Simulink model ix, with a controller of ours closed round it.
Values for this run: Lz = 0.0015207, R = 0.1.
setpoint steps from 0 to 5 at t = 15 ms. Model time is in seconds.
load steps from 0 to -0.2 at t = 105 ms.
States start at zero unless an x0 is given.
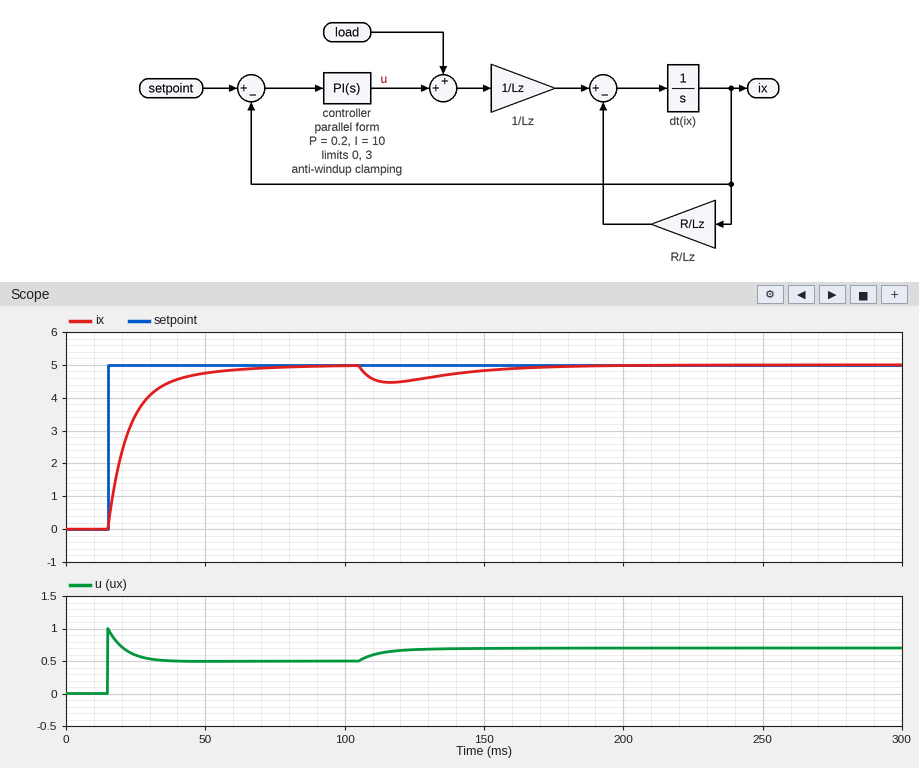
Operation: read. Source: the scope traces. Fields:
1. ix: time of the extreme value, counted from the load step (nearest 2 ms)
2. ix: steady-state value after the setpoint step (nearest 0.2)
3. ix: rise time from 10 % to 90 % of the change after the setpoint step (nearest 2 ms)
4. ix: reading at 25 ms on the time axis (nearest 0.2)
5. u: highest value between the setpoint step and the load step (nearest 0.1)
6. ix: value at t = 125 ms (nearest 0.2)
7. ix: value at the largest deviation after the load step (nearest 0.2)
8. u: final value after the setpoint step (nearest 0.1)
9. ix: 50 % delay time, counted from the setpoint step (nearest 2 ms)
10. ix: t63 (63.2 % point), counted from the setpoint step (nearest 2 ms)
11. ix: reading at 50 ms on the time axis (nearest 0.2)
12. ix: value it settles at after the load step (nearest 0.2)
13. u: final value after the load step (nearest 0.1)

12 ms
5.0
22 ms
3.4
1.0
4.6
4.4
0.5
6 ms
8 ms
4.8
5.0
0.7
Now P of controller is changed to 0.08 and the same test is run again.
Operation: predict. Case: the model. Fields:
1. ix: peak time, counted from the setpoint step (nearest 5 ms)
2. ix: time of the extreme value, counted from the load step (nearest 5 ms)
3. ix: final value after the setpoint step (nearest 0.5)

45 ms
15 ms
5.0
